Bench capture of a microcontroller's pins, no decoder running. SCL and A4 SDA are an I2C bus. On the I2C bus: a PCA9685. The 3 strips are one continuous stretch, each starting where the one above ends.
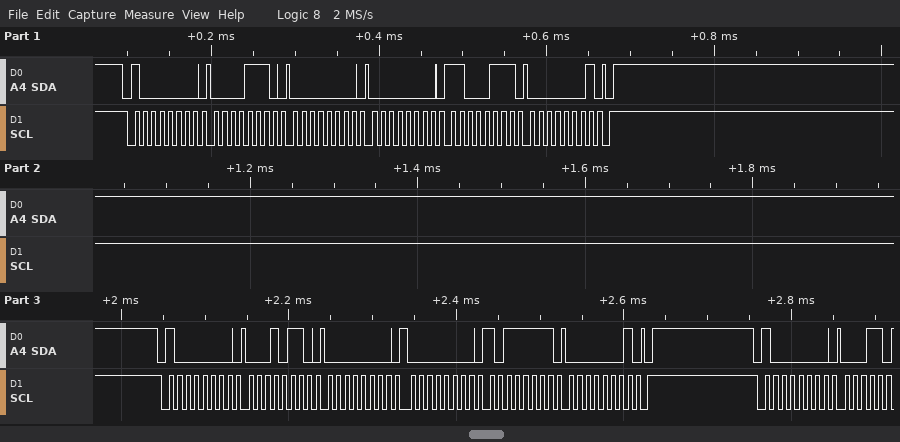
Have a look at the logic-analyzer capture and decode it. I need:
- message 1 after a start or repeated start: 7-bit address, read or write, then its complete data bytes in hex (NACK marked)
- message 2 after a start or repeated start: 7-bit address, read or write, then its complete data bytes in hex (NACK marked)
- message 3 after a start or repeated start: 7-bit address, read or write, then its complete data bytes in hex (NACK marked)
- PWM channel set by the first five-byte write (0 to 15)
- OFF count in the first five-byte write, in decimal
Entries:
0x40 write: 0E 00 00 C7 01
0x40 write: 16 00 00 BF 01
0x40 write
2
455
